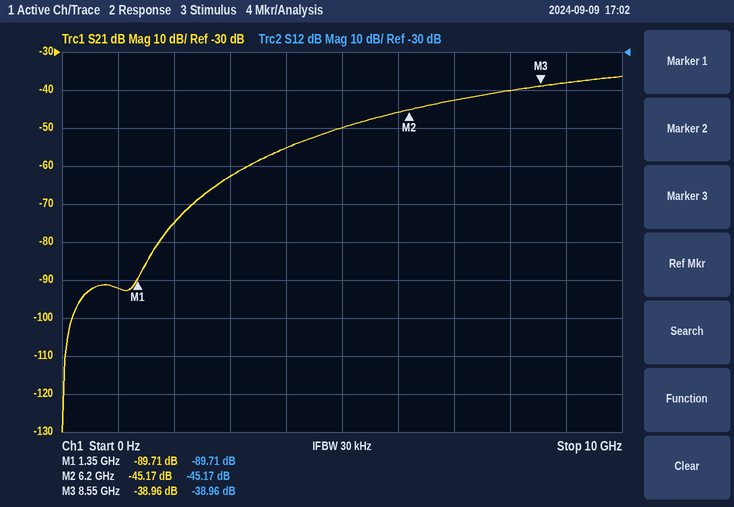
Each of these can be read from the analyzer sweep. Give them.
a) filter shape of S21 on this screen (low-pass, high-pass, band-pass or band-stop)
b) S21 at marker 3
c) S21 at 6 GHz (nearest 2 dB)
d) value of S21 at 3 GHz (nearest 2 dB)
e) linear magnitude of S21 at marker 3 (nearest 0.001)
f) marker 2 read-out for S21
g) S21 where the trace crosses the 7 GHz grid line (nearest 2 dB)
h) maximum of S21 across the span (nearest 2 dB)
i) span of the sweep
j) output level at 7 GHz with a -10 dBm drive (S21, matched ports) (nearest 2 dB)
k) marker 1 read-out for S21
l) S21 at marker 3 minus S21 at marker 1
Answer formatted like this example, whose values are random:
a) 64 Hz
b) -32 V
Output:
a) high-pass
b) -38.96 dB
c) -46 dB
d) -62 dB
e) 0.011
f) -45.17 dB
g) -42 dB
h) -36 dB
i) 10 GHz
j) -52 dBm
k) -89.71 dB
l) 50.75 dB
